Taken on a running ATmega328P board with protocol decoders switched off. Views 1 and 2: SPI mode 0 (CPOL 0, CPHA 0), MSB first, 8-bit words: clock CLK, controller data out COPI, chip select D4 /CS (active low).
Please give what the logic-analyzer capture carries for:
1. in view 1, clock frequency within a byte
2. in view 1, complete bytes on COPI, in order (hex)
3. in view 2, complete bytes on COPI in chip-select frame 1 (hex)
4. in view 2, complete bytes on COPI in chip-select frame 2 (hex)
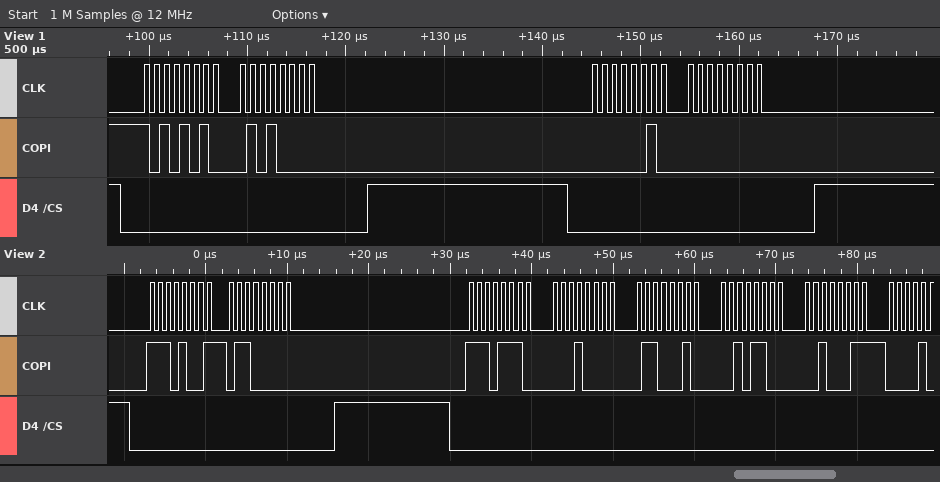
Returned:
1 MHz
AA 50 02 00
E9 60
EE 10 62 2C 23
